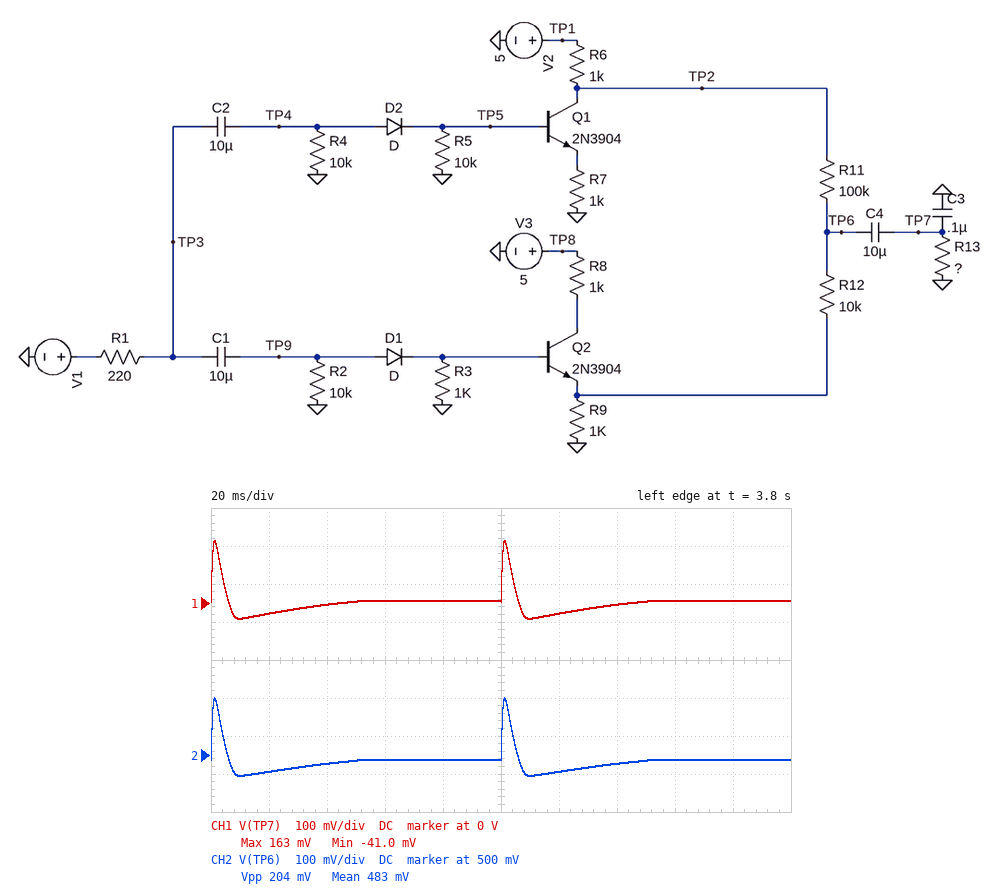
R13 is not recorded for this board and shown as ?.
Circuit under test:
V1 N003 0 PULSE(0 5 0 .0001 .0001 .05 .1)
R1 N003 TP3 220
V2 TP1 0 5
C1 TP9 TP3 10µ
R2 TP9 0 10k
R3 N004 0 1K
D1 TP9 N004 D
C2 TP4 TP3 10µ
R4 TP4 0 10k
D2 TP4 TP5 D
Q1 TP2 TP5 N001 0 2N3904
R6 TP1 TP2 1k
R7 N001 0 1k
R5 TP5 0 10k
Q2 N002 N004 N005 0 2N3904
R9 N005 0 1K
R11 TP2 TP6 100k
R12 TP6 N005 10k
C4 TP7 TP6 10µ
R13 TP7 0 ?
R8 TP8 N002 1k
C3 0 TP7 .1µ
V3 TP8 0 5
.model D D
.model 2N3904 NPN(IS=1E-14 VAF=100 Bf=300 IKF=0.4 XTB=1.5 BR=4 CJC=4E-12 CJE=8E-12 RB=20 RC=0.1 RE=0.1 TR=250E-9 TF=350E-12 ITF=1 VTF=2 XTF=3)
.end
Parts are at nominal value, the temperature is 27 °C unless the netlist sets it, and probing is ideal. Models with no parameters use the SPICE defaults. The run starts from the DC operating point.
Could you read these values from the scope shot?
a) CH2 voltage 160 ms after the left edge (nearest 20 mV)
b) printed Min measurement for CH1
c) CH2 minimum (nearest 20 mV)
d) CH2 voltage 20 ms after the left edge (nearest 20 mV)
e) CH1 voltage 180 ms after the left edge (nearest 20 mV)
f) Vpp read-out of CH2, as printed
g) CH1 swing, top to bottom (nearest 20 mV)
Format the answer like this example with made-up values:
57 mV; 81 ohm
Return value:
480 mV; -41.0 mV; 440 mV; 460 mV; 0 V; 204 mV; 200 mV
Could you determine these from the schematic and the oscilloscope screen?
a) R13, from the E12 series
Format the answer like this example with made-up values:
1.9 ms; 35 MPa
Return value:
12 kΩ
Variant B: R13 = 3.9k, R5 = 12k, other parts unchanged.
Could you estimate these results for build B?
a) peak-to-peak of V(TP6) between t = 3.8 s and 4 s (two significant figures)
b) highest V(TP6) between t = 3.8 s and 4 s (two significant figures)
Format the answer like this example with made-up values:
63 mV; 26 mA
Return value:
120 mV; 580 mV
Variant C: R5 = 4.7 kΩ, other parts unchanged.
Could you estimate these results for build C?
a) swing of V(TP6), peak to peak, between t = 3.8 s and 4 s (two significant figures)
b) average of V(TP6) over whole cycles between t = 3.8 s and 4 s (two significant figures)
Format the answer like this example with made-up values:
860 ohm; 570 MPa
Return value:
190 mV; 490 mV
